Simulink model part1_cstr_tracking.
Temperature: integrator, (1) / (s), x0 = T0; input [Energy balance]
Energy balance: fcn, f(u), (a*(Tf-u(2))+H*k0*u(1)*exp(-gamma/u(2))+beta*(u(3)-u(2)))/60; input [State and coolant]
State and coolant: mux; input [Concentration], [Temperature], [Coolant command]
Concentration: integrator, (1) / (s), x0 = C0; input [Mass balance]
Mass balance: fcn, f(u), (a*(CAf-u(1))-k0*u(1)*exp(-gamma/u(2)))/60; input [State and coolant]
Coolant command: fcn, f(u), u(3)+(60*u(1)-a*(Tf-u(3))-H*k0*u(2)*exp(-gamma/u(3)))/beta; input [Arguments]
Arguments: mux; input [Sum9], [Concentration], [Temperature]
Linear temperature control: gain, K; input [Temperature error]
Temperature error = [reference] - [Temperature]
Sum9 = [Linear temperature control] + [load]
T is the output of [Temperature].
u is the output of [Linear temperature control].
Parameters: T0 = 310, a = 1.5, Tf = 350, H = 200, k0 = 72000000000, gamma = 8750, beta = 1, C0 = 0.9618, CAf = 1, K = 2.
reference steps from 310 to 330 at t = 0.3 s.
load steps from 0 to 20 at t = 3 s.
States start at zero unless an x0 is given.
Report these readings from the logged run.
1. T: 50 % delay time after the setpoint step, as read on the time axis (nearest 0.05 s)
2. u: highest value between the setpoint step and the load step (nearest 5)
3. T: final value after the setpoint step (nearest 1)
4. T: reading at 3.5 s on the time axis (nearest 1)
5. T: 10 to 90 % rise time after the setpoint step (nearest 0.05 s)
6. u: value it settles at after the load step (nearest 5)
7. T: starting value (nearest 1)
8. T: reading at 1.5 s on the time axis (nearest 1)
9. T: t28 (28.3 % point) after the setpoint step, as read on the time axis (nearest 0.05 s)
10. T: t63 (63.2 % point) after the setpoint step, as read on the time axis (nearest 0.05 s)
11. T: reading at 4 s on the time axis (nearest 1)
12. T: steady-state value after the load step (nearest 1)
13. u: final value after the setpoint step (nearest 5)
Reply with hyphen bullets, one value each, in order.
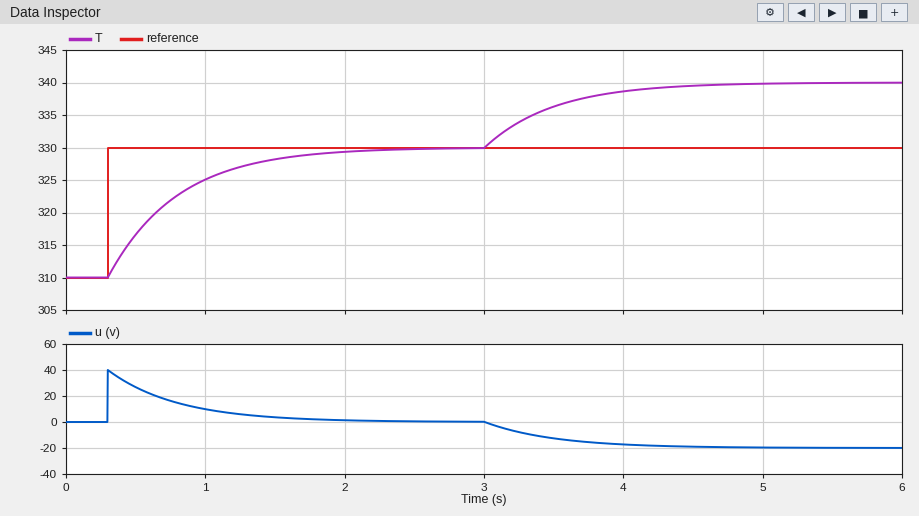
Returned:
- 0.65 s
- 40
- 330
- 336
- 1.10 s
- -20
- 310
- 328
- 0.45 s
- 0.80 s
- 339
- 340
- 0
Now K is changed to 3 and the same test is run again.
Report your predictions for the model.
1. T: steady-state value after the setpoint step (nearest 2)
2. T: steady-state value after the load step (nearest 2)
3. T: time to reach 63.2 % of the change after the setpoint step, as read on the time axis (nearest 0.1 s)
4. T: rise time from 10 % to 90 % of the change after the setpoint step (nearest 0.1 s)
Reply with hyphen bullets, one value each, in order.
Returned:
- 330
- 336
- 0.6 s
- 0.7 s
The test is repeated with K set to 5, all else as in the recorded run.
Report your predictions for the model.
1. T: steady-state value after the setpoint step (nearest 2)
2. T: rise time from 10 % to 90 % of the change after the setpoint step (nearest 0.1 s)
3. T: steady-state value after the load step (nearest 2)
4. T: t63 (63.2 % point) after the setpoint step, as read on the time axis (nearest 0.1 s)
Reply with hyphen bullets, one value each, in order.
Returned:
- 330
- 0.4 s
- 334
- 0.5 s
